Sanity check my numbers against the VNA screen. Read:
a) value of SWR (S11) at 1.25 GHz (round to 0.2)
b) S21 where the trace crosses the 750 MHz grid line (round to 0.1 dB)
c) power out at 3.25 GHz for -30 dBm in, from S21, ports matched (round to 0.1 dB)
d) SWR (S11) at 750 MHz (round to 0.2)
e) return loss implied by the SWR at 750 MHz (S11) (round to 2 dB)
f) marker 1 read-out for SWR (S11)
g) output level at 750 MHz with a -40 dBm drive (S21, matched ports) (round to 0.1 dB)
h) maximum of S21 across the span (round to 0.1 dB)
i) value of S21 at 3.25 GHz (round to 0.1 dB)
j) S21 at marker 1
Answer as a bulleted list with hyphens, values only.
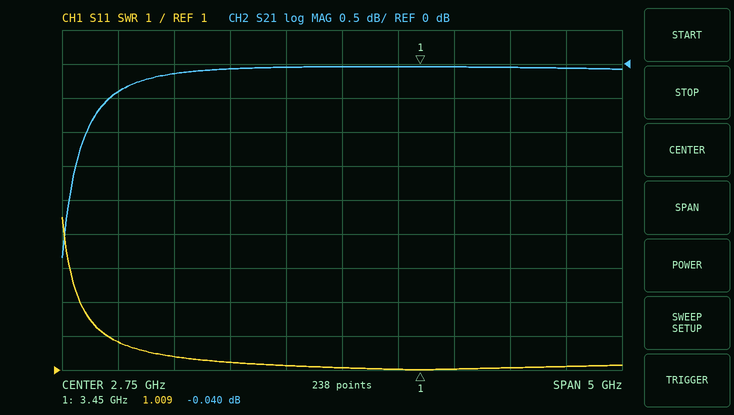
- 1.4
- -0.4 dB
- -30.0 dBm
- 1.8
- 10 dB
- 1.009
- -40.4 dBm
- 0.0 dB
- 0.0 dB
- -0.040 dB
